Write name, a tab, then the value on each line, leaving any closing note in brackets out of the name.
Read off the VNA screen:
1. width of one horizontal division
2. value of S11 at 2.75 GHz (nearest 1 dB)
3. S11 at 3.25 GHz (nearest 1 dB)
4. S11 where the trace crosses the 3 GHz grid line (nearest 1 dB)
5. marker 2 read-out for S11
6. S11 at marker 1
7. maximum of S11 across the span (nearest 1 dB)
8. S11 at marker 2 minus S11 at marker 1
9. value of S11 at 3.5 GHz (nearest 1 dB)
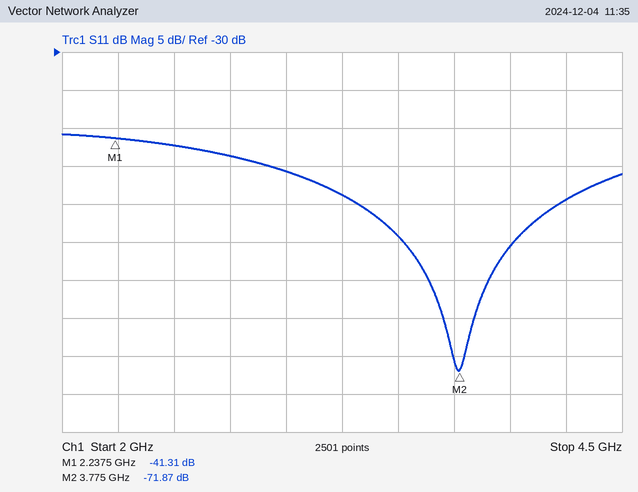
width of one horizontal division	250 MHz
value of S11 at 2.75 GHz	-44 dB
S11 at 3.25 GHz	-49 dB
S11 where the trace crosses the 3 GHz grid line	-46 dB
marker 2 read-out for S11	-71.87 dB
S11 at marker 1	-41.31 dB
maximum of S11 across the span	-41 dB
S11 at marker 2 minus S11 at marker 1	-30.56 dB
value of S11 at 3.5 GHz	-54 dB
